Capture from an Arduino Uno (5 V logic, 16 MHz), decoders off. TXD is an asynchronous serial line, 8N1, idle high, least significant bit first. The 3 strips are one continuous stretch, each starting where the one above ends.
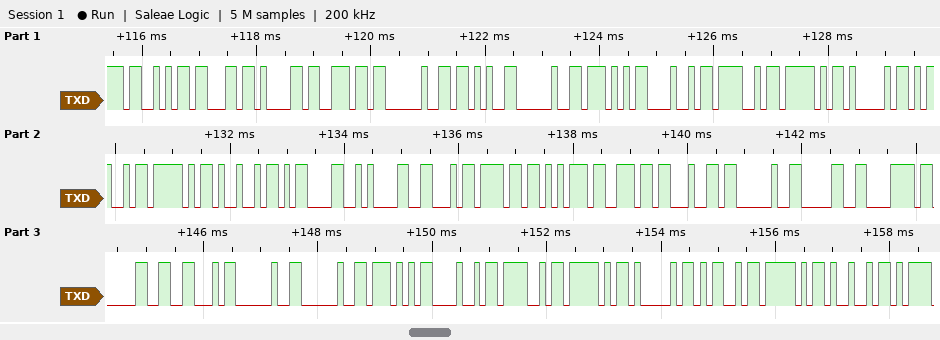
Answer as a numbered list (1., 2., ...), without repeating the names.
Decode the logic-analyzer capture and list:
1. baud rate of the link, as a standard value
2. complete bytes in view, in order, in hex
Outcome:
1. 9600 baud
2. 53 63 61 6E 20 2B 20 57 48 4F 5F 41 4D 5F 49 0D 0A 46 6F 75 6E 64 20 30 78 30 46 20 20 57 48 4F 5F 41 4D 5F 49
